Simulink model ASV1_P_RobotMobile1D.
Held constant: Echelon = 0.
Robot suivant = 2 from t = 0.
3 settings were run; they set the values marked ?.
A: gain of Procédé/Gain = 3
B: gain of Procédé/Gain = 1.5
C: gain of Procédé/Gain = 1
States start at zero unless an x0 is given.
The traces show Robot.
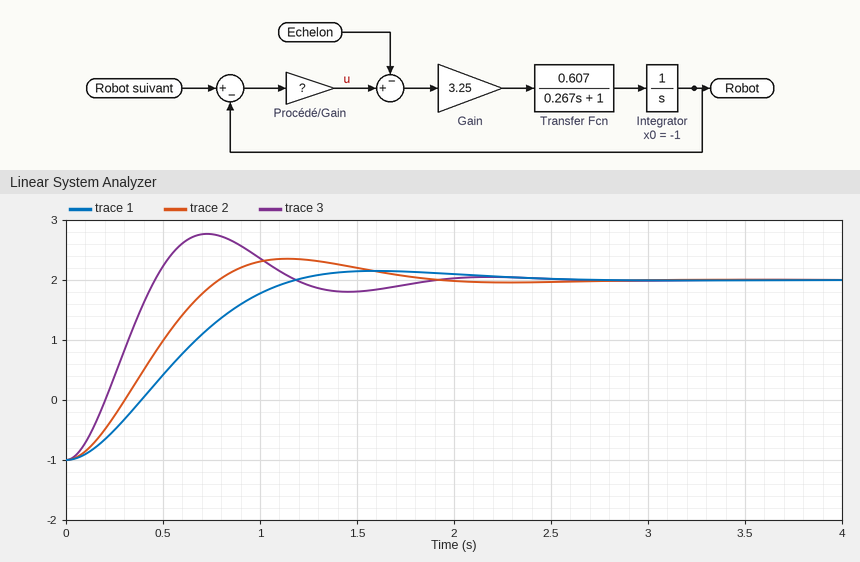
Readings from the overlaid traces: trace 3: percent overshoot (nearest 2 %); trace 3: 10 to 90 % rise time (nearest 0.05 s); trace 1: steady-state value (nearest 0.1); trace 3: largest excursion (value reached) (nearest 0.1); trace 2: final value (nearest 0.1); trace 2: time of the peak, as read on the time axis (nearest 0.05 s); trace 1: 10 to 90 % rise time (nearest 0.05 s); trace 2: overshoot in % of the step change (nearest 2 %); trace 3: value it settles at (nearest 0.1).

26 %
0.30 s
2.0
2.8
2.0
1.15 s
0.75 s
12 %
2.0
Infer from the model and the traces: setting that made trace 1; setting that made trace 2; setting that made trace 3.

C
B
A
